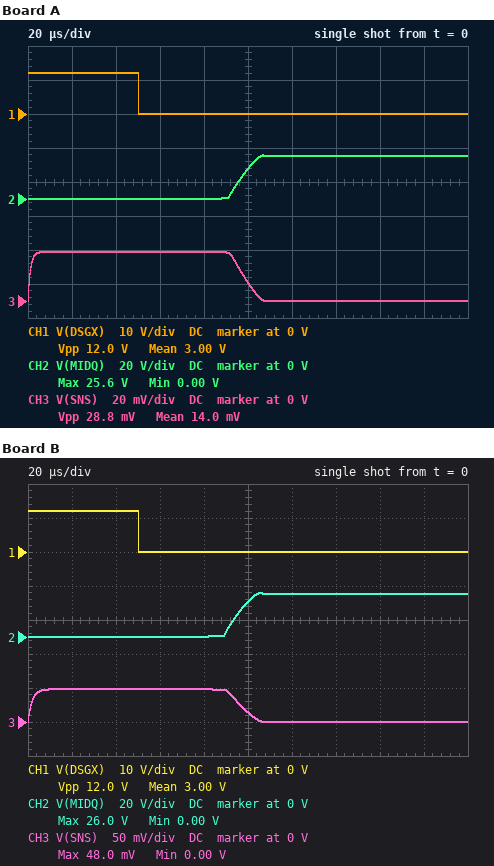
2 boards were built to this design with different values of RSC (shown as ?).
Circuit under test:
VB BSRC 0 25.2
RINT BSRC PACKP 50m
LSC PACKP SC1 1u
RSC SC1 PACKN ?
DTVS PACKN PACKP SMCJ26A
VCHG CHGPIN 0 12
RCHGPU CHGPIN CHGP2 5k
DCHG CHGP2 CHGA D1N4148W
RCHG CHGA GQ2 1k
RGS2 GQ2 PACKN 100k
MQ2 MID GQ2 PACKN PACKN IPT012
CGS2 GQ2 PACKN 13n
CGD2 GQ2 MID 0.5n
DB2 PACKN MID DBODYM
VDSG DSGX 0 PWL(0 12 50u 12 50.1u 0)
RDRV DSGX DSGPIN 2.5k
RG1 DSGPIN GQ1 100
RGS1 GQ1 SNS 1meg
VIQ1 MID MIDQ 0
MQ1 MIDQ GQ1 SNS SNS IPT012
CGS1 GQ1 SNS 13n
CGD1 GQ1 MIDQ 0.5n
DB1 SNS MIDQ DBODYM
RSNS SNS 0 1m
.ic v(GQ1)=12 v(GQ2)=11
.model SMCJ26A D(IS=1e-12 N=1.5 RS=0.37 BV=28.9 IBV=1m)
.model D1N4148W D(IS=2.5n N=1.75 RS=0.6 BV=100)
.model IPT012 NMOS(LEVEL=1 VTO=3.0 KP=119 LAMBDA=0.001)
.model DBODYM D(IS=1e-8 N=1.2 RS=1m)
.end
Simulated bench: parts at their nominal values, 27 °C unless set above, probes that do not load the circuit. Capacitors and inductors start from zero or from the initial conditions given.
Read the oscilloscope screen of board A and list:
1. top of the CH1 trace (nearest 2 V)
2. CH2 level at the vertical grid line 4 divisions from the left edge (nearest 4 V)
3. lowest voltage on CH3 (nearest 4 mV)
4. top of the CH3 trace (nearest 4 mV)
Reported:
12 V
0 V
0 V
28 mV
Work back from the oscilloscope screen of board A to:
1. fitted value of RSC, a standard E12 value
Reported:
0.82 Ω
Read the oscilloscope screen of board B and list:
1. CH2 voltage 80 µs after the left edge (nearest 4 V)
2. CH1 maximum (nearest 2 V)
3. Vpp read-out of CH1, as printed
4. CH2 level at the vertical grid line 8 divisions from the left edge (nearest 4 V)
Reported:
0 V
12 V
12.0 V
24 V
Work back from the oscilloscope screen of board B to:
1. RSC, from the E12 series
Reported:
0.47 Ω
